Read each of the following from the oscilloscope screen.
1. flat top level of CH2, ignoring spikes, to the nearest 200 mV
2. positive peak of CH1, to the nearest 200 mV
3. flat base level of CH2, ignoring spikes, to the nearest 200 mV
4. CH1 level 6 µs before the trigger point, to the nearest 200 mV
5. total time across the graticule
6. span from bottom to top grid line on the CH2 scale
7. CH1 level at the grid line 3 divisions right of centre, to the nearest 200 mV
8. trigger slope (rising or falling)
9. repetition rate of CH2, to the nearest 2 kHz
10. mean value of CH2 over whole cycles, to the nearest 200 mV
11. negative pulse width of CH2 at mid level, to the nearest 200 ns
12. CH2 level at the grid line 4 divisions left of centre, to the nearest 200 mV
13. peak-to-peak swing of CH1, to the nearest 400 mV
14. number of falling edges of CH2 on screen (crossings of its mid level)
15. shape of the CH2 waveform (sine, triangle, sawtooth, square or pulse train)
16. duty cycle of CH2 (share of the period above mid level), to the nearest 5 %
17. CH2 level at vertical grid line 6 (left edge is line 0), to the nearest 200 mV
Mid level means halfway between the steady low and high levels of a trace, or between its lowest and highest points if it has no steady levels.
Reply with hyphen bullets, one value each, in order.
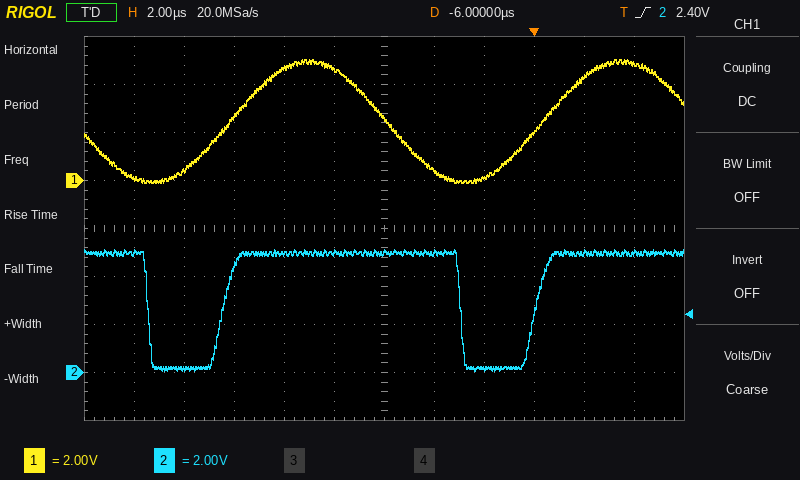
- 5.0 V
- 5.0 V
- 200 mV
- 2.6 V
- 24 µs
- 16 V
- 2.0 V
- rising
- 80 kHz
- 3.8 V
- 3.0 µs
- 200 mV
- 5.2 V
- 2
- pulse train
- 75 %
- 5.0 V
